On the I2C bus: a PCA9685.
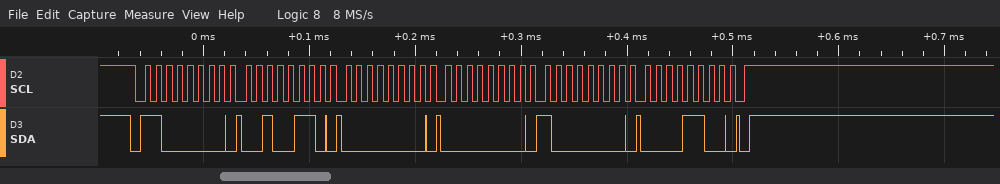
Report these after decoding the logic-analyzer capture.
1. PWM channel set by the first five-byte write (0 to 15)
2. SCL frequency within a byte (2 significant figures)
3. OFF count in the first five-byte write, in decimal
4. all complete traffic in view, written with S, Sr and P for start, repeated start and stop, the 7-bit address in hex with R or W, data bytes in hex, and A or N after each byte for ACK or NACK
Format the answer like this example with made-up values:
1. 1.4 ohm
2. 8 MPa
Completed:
1. 8
2. 100 kHz
3. 3200
4. S 60W A 26 A 00 A 00 A 80 A 0C A P
